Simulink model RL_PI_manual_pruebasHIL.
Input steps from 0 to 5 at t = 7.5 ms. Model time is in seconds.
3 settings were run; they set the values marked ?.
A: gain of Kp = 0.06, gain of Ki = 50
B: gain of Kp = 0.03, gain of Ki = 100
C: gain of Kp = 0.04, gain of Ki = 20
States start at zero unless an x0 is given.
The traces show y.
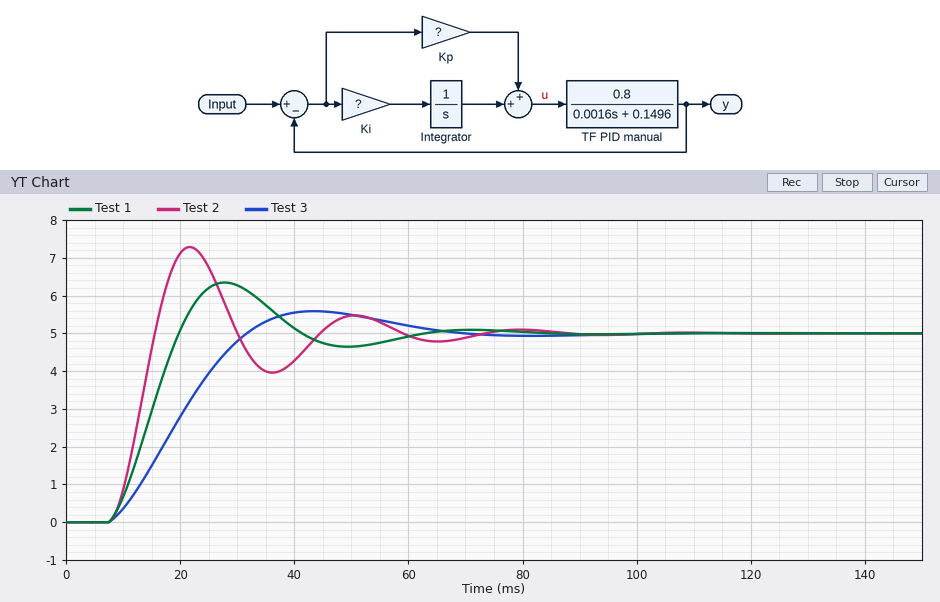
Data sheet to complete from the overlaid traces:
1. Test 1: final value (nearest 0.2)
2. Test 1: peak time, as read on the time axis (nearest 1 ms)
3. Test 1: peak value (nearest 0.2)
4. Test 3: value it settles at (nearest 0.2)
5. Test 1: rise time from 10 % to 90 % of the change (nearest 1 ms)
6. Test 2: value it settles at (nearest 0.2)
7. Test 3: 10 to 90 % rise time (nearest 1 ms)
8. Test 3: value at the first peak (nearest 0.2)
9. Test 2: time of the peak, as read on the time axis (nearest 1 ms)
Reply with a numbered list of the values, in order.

1. 5.0
2. 28 ms
3. 6.4
4. 5.0
5. 9 ms
6. 5.0
7. 17 ms
8. 5.6
9. 22 ms
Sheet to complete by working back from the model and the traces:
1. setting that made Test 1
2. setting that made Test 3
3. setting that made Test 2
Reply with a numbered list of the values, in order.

1. A
2. C
3. B
